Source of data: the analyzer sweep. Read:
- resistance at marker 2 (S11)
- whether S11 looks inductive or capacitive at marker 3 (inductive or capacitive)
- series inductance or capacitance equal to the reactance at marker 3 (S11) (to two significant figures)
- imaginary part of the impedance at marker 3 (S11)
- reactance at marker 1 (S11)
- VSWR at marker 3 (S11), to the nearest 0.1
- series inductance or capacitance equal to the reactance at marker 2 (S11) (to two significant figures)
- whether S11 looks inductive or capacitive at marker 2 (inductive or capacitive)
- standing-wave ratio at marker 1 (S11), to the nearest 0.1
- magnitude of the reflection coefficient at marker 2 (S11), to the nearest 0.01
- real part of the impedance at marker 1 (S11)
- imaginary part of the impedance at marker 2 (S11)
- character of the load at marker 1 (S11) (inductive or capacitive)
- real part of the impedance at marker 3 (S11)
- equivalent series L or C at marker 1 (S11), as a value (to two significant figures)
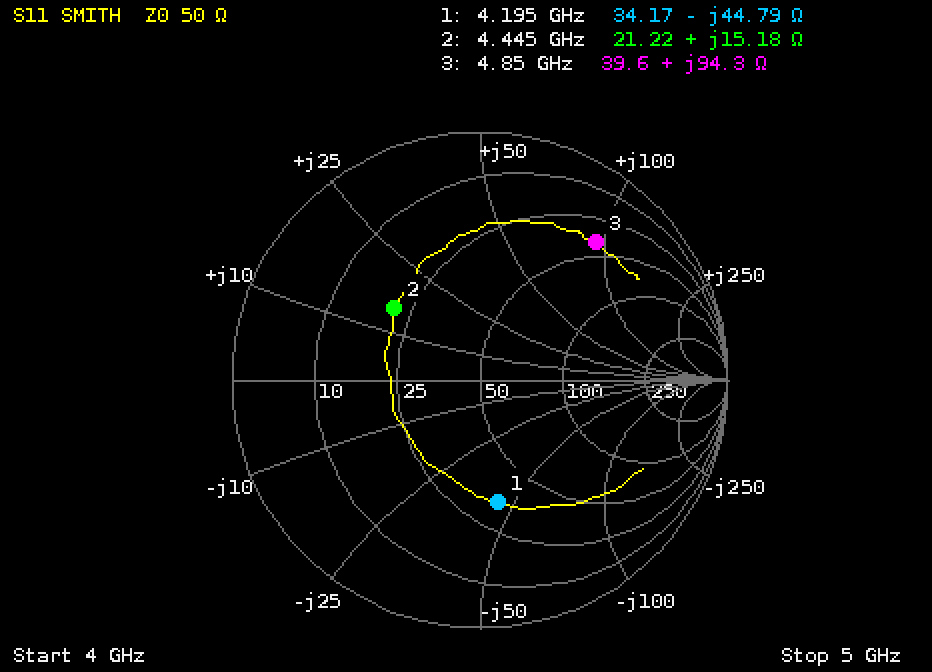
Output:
21.22 Ω
inductive
3.1 nH
+94.3 Ω
-44.79 Ω
6.4
540 pH
inductive
3.0
0.45
34.17 Ω
+15.18 Ω
capacitive
39.6 Ω
850 fF
